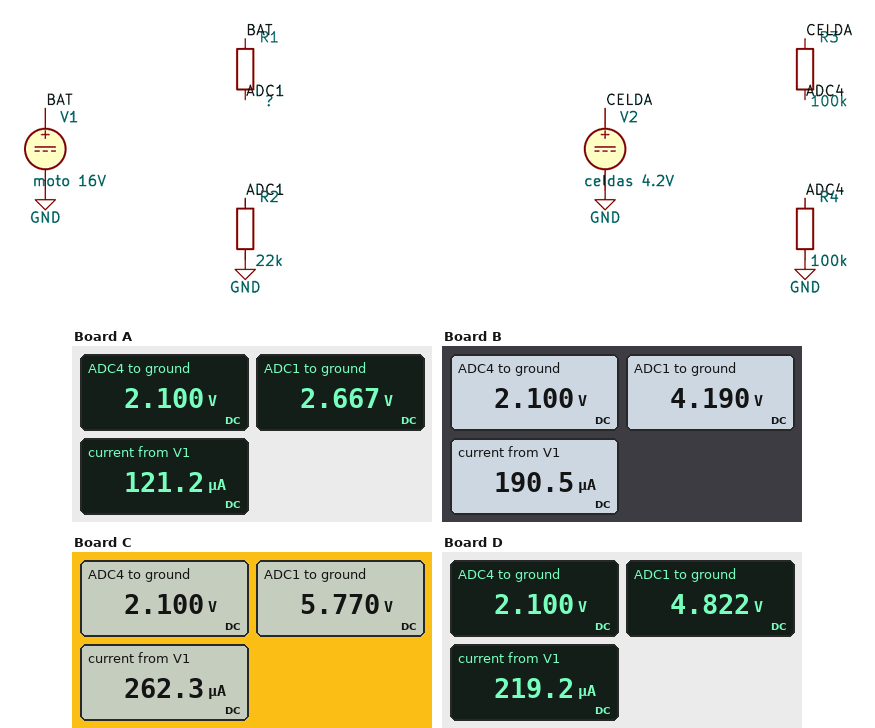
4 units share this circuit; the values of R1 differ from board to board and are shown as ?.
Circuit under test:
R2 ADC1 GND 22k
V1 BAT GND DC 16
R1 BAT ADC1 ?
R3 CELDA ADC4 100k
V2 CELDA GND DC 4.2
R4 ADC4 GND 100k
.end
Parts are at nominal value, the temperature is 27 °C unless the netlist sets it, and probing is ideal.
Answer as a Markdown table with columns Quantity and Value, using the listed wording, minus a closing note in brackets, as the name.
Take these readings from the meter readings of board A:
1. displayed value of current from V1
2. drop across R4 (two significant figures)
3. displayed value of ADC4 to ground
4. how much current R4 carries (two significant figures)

| Quantity | Value |
|---|---|
| displayed value of current from V1 | 121.2 µA |
| drop across R4 | 2.1 V |
| displayed value of ADC4 to ground | 2.100 V |
| how much current R4 carries | 21 µA |
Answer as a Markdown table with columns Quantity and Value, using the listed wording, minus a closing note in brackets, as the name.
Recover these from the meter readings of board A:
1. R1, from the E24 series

| Quantity | Value |
|---|---|
| R1, from the E24 series | 110 kΩ |
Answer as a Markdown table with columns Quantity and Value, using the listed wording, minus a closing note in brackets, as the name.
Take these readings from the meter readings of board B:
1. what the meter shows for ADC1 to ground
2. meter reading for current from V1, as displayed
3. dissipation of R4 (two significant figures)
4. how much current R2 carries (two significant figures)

| Quantity | Value |
|---|---|
| what the meter shows for ADC1 to ground | 4.190 V |
| meter reading for current from V1, as displayed | 190.5 µA |
| dissipation of R4 | 44 µW |
| how much current R2 carries | 190 µA |
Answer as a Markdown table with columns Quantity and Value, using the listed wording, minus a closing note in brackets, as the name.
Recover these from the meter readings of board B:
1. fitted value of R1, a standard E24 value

| Quantity | Value |
|---|---|
| fitted value of R1, a standard E24 value | 62 kΩ |
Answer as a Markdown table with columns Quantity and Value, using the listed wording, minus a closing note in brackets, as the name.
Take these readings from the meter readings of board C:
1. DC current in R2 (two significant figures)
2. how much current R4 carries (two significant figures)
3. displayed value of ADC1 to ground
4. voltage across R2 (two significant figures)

| Quantity | Value |
|---|---|
| DC current in R2 | 260 µA |
| how much current R4 carries | 21 µA |
| displayed value of ADC1 to ground | 5.770 V |
| voltage across R2 | 5.8 V |
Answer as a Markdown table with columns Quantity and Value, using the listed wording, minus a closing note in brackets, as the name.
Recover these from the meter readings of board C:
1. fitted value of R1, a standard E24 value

| Quantity | Value |
|---|---|
| fitted value of R1, a standard E24 value | 39 kΩ |
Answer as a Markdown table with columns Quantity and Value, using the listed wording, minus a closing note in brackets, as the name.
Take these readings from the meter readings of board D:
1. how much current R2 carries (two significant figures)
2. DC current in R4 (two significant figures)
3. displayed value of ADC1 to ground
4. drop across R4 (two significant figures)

| Quantity | Value |
|---|---|
| how much current R2 carries | 220 µA |
| DC current in R4 | 21 µA |
| displayed value of ADC1 to ground | 4.822 V |
| drop across R4 | 2.1 V |
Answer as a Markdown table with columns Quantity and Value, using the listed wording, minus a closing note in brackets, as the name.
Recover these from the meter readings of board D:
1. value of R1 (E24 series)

| Quantity | Value |
|---|---|
| value of R1 | 51 kΩ |
